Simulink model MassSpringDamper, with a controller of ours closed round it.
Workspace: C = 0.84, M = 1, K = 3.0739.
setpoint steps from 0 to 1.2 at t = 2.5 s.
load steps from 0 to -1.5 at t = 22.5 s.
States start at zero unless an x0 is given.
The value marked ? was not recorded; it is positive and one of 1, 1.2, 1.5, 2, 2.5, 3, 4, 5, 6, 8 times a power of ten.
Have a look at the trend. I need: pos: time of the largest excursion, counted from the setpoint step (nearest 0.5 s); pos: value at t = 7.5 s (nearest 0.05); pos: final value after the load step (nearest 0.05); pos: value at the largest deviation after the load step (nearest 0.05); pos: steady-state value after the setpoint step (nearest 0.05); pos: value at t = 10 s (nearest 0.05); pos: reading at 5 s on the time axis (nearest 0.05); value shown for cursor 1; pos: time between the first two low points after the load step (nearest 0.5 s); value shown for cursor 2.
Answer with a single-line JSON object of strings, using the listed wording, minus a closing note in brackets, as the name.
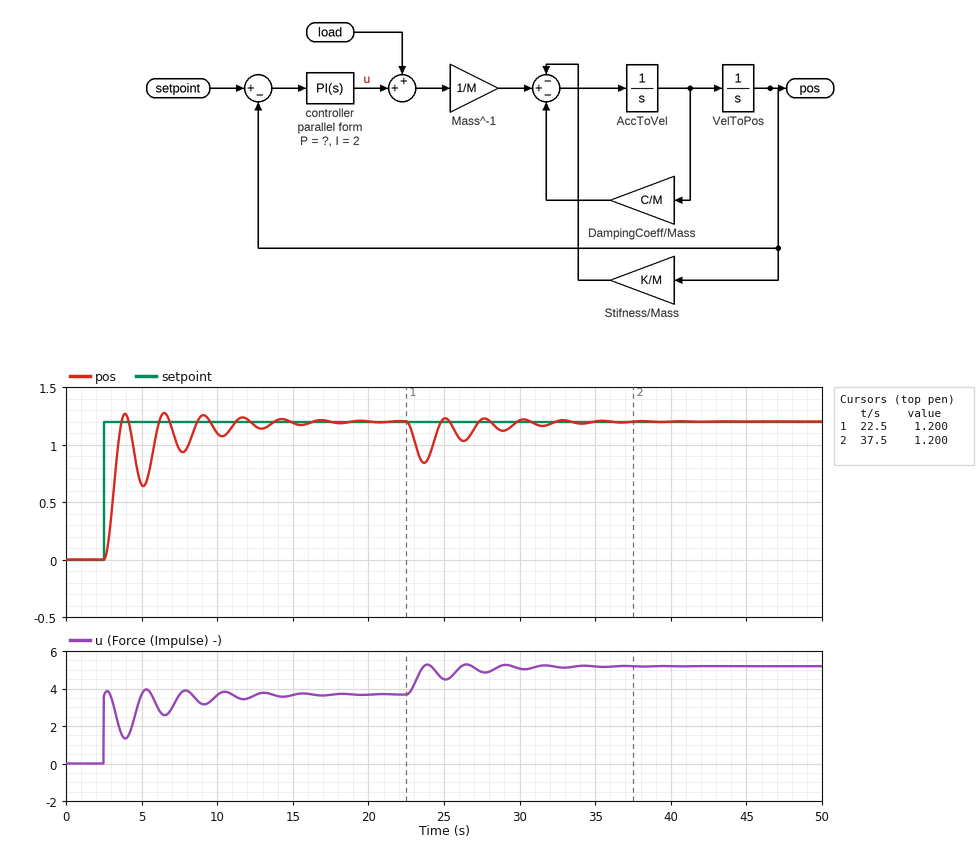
{"pos: time of the largest excursion, counted from the setpoint step": "4.0 s", "pos: value at t = 7.5 s": "0.95", "pos: final value after the load step": "1.20", "pos: value at the largest deviation after the load step": "0.85", "pos: steady-state value after the setpoint step": "1.20", "pos: value at t = 10 s": "1.10", "pos: reading at 5 s on the time axis": "0.65", "value shown for cursor 1": "1.200", "pos: time between the first two low points after the load step": "2.5 s", "value shown for cursor 2": "1.200"}
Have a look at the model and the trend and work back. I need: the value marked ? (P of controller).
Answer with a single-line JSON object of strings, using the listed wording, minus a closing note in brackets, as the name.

{"the value marked ?": "3"}
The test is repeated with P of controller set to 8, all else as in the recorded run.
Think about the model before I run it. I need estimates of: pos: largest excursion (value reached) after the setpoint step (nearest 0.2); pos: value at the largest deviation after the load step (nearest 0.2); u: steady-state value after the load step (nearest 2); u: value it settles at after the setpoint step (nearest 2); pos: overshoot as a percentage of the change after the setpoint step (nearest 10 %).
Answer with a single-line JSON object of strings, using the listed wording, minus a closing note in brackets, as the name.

{"pos: largest excursion (value reached) after the setpoint step": "1.6", "pos: value at the largest deviation after the load step": "1.0", "u: steady-state value after the load step": "6", "u: value it settles at after the setpoint step": "4", "pos: overshoot as a percentage of the change after the setpoint step": "30 %"}
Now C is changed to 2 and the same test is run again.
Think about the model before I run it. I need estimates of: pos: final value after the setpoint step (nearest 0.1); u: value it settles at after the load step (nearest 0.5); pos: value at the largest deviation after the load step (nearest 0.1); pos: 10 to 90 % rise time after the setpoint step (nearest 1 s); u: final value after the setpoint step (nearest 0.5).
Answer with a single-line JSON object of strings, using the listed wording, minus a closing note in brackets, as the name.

{"pos: final value after the setpoint step": "1.2", "u: value it settles at after the load step": "5.0", "pos: value at the largest deviation after the load step": "0.9", "pos: 10 to 90 % rise time after the setpoint step": "4 s", "u: final value after the setpoint step": "3.5"}
